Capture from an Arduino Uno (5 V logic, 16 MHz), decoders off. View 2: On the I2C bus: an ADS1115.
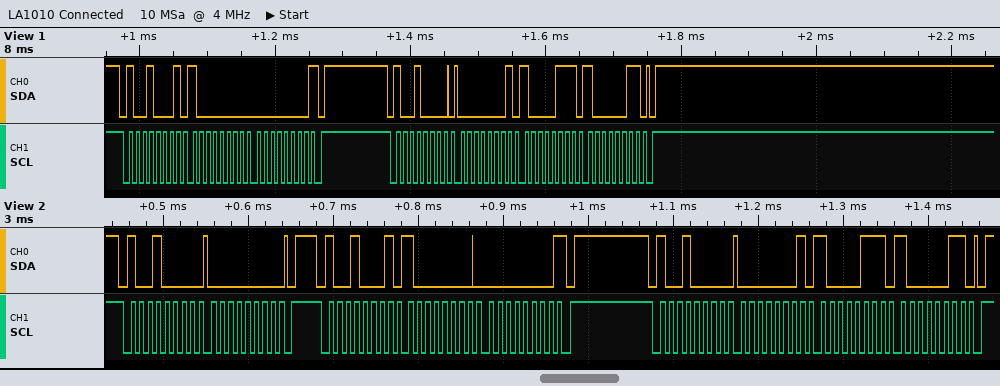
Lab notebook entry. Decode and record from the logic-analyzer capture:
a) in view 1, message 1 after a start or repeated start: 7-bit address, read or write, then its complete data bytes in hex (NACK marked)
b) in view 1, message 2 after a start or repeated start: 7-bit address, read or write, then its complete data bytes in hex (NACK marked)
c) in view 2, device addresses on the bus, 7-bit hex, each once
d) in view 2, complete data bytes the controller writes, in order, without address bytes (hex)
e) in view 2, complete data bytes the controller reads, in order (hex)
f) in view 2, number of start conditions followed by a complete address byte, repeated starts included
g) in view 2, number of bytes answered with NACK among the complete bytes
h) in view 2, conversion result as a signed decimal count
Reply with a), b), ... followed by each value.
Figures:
a) 0x48 read: 80 00 NACK
b) 0x48 write: 01 87 83
c) 0x48
d) 00 01 87 83
e) 80 00
f) 3
g) 1
h) -32768
